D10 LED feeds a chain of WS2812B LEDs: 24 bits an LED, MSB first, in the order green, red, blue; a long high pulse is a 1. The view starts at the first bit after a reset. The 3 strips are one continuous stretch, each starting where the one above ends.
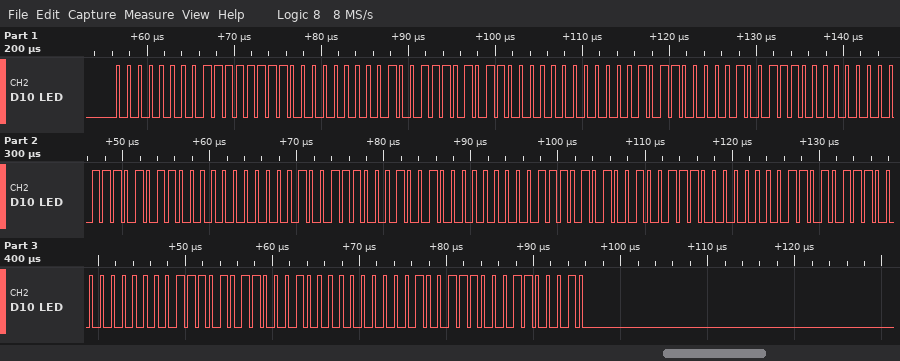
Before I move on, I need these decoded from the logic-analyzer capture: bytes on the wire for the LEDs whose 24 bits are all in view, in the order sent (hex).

00 FF 00 4E B0 00 B0 4E 00 EB 00 13 89 00 75 27 00 D7 00 3A C4 00 9C 62
